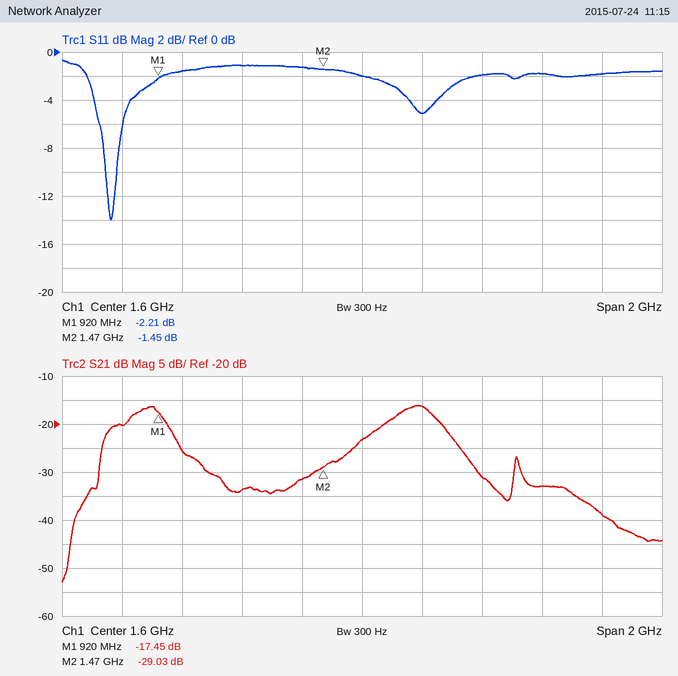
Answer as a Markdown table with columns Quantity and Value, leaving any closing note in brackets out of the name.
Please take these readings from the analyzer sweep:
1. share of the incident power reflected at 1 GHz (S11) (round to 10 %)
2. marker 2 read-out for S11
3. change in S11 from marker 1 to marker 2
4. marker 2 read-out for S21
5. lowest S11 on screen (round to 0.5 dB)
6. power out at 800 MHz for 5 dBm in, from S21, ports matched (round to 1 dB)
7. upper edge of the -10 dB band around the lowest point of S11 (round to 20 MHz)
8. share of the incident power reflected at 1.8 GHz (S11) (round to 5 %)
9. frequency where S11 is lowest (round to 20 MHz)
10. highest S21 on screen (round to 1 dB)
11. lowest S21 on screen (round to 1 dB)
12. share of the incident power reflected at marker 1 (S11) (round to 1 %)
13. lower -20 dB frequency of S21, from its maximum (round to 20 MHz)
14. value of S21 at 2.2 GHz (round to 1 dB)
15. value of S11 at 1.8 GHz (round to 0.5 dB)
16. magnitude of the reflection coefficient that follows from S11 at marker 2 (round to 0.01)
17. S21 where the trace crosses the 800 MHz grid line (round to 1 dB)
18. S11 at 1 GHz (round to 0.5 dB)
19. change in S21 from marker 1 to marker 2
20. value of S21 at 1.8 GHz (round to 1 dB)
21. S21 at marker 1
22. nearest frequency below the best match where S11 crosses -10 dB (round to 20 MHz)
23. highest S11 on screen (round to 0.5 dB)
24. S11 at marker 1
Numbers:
| Quantity | Value |
|---|---|
| share of the incident power reflected at 1 GHz (S11) | 70 % |
| marker 2 read-out for S11 | -1.45 dB |
| change in S11 from marker 1 to marker 2 | 0.76 dB |
| marker 2 read-out for S21 | -29.03 dB |
| lowest S11 on screen | -14.0 dB |
| power out at 800 MHz for 5 dBm in, from S21, ports matched | -15 dBm |
| upper edge of the -10 dB band around the lowest point of S11 | 780 MHz |
| share of the incident power reflected at 1.8 GHz (S11) | 30 % |
| frequency where S11 is lowest | 760 MHz |
| highest S21 on screen | -16 dB |
| lowest S21 on screen | -53 dB |
| share of the incident power reflected at marker 1 (S11) | 60 % |
| lower -20 dB frequency of S21, from its maximum | 680 MHz |
| value of S21 at 2.2 GHz | -33 dB |
| value of S11 at 1.8 GHz | -5.0 dB |
| magnitude of the reflection coefficient that follows from S11 at marker 2 | 0.85 |
| S21 where the trace crosses the 800 MHz grid line | -20 dB |
| S11 at 1 GHz | -1.5 dB |
| change in S21 from marker 1 to marker 2 | -11.58 dB |
| value of S21 at 1.8 GHz | -16 dB |
| S21 at marker 1 | -17.45 dB |
| nearest frequency below the best match where S11 crosses -10 dB | 740 MHz |
| highest S11 on screen | -0.5 dB |
| S11 at marker 1 | -2.21 dB |
